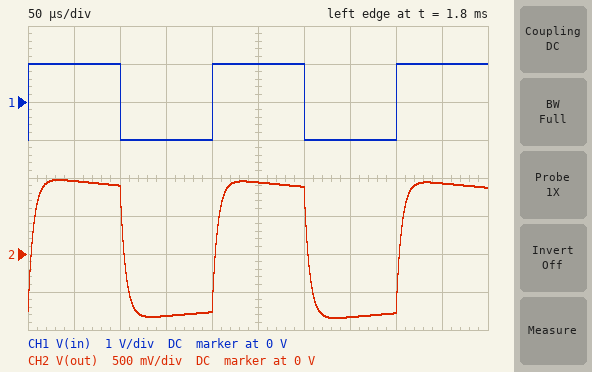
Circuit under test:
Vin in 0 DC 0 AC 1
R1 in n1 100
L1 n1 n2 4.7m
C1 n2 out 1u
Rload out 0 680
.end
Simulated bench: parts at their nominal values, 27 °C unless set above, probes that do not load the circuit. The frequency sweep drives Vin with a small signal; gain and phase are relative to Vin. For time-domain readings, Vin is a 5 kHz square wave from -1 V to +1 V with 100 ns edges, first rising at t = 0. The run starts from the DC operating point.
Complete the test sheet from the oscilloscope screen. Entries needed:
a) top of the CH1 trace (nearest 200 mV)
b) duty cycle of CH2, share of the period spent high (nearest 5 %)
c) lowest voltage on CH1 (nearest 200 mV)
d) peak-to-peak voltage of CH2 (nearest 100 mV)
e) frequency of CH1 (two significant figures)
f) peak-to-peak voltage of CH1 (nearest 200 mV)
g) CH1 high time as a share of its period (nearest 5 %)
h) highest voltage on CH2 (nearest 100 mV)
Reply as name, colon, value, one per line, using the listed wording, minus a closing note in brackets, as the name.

top of the CH1 trace: 1.0 V
duty cycle of CH2, share of the period spent high: 50 %
lowest voltage on CH1: -1.0 V
peak-to-peak voltage of CH2: 1.8 V
frequency of CH1: 5.0 kHz
peak-to-peak voltage of CH1: 2.0 V
CH1 high time as a share of its period: 50 %
highest voltage on CH2: 1.0 V
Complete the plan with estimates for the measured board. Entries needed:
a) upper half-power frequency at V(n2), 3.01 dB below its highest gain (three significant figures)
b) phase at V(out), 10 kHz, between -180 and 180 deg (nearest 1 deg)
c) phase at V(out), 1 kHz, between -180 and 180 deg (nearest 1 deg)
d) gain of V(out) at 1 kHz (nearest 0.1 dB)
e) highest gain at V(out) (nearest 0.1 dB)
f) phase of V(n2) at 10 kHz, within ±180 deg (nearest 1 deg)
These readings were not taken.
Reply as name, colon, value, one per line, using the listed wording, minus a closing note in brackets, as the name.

upper half-power frequency at V(n2), 3.01 dB below its highest gain: 19.3 kHz
phase at V(out), 10 kHz, between -180 and 180 deg: -20 deg
phase at V(out), 1 kHz, between -180 and 180 deg: 9 deg
gain of V(out) at 1 kHz: -1.3 dB
highest gain at V(out): -1.2 dB
phase of V(n2) at 10 kHz, within ±180 deg: -21 deg
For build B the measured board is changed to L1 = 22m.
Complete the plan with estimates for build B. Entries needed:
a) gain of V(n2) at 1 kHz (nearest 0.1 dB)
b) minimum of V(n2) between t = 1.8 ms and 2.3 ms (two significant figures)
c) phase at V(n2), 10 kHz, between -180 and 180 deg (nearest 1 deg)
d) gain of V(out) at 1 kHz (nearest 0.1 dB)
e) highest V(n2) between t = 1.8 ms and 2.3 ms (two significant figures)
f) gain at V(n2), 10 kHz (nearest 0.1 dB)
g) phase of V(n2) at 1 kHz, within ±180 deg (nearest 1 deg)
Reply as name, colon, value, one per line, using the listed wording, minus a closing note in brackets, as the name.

gain of V(n2) at 1 kHz: -1.0 dB
minimum of V(n2) between t = 1.8 ms and 2.3 ms: -860 mV
phase at V(n2), 10 kHz, between -180 and 180 deg: -62 deg
gain of V(out) at 1 kHz: -1.2 dB
highest V(n2) between t = 1.8 ms and 2.3 ms: 850 mV
gain at V(n2), 10 kHz: -7.3 dB
phase of V(n2) at 1 kHz, within ±180 deg: -12 deg
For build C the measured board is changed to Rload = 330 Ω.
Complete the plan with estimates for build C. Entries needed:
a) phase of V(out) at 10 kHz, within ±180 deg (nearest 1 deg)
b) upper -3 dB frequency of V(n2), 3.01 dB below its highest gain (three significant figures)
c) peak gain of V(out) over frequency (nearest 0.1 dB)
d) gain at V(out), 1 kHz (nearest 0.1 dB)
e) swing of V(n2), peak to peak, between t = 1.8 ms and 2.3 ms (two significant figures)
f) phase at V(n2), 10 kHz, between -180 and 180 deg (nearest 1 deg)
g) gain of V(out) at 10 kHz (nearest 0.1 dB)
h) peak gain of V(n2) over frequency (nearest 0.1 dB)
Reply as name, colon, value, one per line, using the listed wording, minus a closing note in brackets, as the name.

phase of V(out) at 10 kHz, within ±180 deg: -33 deg
upper -3 dB frequency of V(n2), 3.01 dB below its highest gain: 7.01 kHz
peak gain of V(out) over frequency: -2.3 dB
gain at V(out), 1 kHz: -2.7 dB
swing of V(n2), peak to peak, between t = 1.8 ms and 2.3 ms: 1.6 V
phase at V(n2), 10 kHz, between -180 and 180 deg: -36 deg
gain of V(out) at 10 kHz: -3.8 dB
peak gain of V(n2) over frequency: 0 dB
